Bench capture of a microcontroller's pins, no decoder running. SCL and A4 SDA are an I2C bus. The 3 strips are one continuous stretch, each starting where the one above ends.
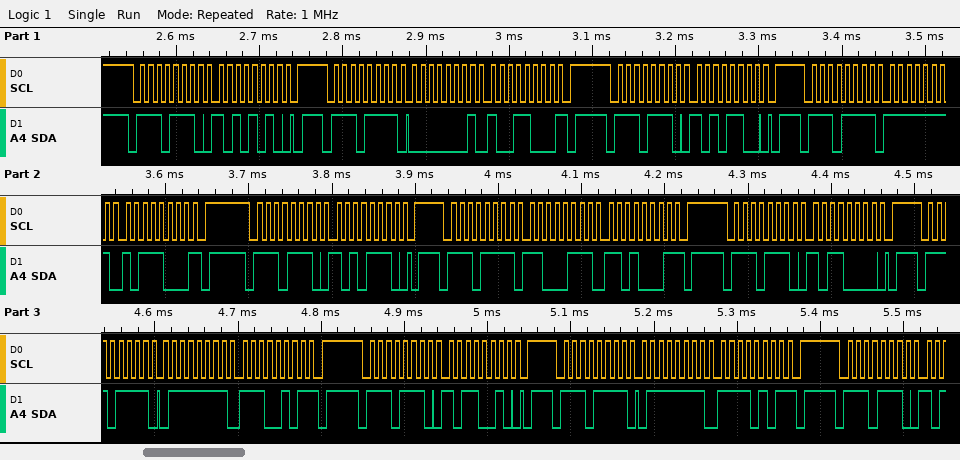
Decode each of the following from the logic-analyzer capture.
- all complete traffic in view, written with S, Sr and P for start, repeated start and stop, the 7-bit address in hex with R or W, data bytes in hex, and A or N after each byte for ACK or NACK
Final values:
S 77W A AA A P S 77R A 01 A 98 N P S 77W A AC A P S 77R A FF A B8 N P S 77W A AE A P S 77R A C7 A D1 N P S 77W A B0 A P S 77R A 7F A E5 N P S 77W A B2 A P S 77R A 7F A F5 N P S 77W A
